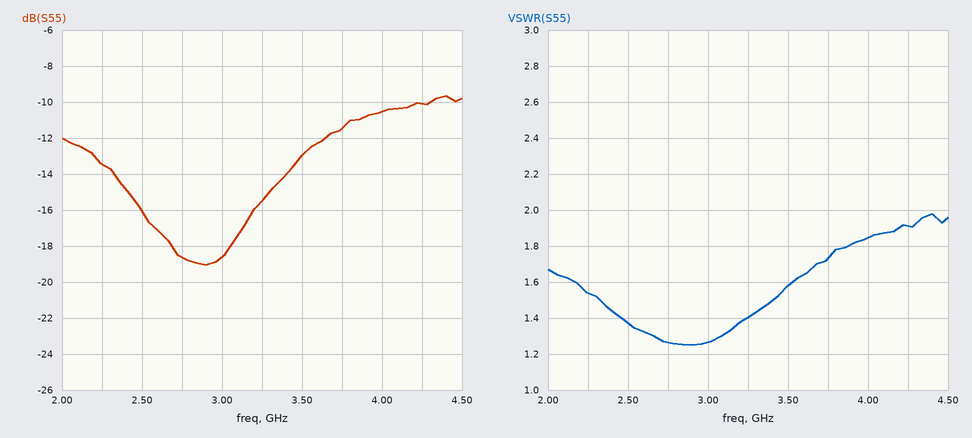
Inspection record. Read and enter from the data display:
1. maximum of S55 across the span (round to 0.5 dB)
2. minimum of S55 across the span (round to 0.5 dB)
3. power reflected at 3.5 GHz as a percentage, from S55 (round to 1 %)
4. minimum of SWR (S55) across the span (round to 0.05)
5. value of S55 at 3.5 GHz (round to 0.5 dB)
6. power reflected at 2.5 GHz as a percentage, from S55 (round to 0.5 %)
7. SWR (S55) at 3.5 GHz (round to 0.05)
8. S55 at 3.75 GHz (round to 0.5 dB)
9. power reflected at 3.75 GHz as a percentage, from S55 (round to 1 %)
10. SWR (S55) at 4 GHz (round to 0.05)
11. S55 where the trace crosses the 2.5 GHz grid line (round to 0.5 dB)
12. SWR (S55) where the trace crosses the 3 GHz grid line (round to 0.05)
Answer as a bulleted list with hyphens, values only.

- -9.5 dB
- -19.0 dB
- 5 %
- 1.25
- -13.0 dB
- 2.5 %
- 1.60
- -11.5 dB
- 7 %
- 1.85
- -16.0 dB
- 1.25
